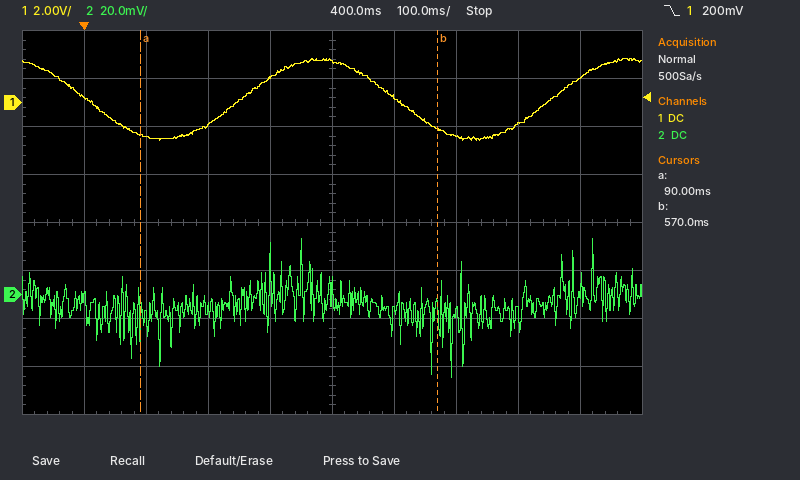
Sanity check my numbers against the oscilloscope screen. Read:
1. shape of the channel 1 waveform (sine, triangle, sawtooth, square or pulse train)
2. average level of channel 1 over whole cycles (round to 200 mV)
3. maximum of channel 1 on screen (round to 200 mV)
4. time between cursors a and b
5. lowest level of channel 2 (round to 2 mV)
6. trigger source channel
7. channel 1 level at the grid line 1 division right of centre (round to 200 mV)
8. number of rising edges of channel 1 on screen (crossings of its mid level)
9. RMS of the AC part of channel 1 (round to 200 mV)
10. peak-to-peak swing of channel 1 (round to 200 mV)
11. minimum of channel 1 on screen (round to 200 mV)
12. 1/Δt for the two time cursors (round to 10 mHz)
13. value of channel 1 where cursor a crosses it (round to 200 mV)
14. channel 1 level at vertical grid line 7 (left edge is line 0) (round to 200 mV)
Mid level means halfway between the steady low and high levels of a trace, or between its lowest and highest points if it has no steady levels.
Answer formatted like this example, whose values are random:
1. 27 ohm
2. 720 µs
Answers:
1. sine
2. 200 mV
3. 1.8 V
4. 480 ms
5. -34 mV
6. channel 1
7. 200 mV
8. 2
9. 1.2 V
10. 3.4 V
11. -1.6 V
12. 2.08 Hz
13. -1.4 V
14. -1.4 V
